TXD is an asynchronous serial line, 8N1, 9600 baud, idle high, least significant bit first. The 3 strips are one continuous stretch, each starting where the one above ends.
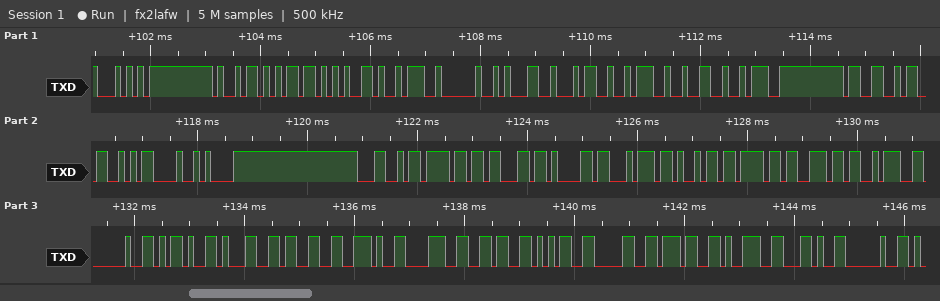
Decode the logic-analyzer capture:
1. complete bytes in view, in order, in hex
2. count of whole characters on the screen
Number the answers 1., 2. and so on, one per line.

1. 54 69 6D 65 3A 20 31 34 3A 32 3A 33 33 0D 0A 4C 6F 63 61 74 69 6F 6E 3A 20 2D 31 33 2E 38 36 35 30 37 39 2C 20
2. 37
